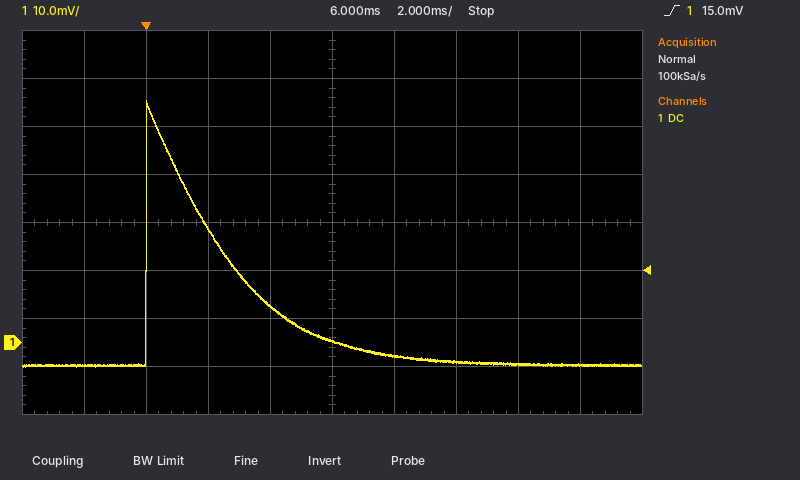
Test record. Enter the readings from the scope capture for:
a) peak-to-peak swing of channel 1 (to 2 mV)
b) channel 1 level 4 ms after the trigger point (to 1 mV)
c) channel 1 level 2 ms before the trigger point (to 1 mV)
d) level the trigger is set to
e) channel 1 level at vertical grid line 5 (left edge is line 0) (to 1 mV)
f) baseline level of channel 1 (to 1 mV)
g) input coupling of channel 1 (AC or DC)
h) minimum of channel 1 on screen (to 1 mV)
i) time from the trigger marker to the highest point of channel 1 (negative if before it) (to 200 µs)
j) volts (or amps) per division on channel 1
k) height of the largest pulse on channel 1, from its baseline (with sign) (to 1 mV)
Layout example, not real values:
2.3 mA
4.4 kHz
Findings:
56 mV
8 mV
-5 mV
15.0 mV
0 mV
-5 mV
DC
-5 mV
0.0 ms
10 mV
+55 mV
